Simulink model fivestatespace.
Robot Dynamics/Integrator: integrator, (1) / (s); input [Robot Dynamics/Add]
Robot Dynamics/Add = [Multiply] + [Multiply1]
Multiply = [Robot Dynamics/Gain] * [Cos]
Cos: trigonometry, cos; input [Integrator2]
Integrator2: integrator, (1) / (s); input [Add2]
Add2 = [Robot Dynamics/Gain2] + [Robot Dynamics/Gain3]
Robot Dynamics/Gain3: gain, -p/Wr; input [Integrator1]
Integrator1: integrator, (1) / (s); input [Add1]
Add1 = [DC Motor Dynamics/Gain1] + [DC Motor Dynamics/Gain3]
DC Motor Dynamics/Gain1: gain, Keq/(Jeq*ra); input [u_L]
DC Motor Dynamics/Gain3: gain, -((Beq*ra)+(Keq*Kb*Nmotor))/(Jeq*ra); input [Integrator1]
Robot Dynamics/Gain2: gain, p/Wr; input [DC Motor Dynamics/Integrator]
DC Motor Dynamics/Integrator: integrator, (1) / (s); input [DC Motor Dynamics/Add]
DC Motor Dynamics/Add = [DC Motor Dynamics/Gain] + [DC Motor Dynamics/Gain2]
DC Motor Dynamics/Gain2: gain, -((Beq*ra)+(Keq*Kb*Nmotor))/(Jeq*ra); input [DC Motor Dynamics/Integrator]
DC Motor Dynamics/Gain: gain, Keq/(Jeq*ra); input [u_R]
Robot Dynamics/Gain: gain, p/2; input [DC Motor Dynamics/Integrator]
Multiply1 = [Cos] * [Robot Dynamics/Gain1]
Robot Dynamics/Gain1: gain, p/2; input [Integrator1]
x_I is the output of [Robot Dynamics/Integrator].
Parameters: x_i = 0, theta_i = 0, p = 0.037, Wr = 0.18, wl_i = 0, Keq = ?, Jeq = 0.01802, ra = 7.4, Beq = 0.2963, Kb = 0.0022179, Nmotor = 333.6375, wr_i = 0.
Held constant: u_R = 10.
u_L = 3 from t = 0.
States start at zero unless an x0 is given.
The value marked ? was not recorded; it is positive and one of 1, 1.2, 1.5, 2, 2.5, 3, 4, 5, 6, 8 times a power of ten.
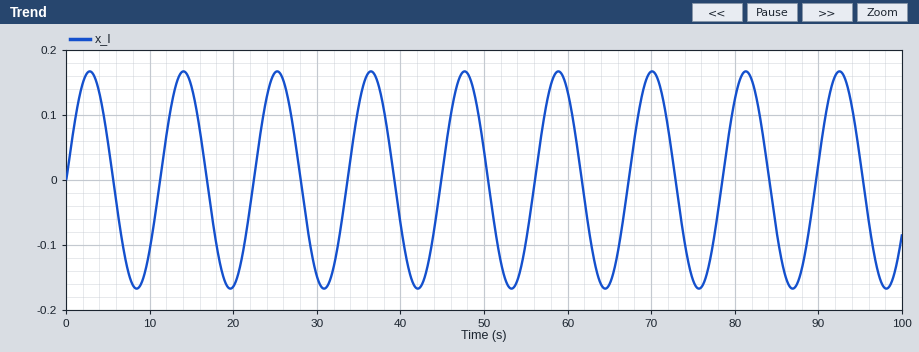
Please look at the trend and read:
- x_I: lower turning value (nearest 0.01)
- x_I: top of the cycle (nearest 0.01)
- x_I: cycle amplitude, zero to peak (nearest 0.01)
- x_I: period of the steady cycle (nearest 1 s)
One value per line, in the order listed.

-0.17
0.17
0.17
11 s
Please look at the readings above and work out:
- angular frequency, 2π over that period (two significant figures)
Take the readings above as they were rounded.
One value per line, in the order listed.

0.57 rad/s
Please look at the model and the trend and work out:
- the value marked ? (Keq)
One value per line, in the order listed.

1.2
